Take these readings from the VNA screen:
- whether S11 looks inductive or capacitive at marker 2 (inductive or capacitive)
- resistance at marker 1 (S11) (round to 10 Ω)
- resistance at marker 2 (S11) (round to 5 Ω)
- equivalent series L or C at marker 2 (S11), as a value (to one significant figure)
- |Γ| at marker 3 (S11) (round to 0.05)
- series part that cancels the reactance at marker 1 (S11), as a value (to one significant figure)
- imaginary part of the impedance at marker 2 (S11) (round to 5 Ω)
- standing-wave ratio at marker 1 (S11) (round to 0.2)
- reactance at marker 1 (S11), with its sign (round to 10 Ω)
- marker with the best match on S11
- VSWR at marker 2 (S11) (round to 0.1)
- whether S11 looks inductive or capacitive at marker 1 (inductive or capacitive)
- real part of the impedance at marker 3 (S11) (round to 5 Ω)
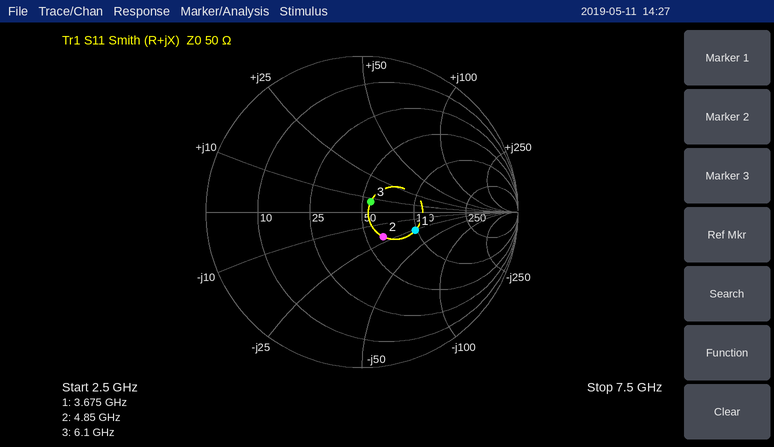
capacitive
100 Ω
60 Ω
2 pF
0.10
1 nH
-20 Ω
2.2
-30 Ω
marker 3
1.5
capacitive
55 Ω
